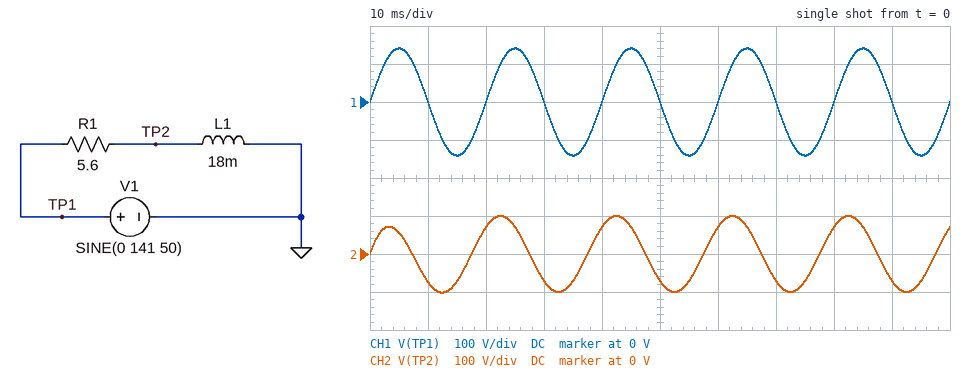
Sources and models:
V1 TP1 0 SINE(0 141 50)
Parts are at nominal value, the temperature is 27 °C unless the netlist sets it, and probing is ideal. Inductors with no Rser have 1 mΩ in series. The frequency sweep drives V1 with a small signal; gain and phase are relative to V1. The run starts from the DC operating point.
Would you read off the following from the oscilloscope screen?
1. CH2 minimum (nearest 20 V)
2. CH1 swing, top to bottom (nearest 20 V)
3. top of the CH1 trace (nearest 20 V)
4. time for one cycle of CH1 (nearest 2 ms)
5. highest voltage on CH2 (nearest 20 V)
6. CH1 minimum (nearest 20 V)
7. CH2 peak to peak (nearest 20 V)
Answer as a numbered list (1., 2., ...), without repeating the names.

1. -100 V
2. 280 V
3. 140 V
4. 20 ms
5. 100 V
6. -140 V
7. 200 V
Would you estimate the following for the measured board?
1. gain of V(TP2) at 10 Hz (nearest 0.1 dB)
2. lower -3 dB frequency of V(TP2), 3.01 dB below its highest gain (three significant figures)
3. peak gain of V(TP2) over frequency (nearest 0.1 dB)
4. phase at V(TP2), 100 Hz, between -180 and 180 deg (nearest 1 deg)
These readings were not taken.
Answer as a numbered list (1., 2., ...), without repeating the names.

1. -14.1 dB
2. 49.5 Hz
3. 0 dB
4. 26 deg
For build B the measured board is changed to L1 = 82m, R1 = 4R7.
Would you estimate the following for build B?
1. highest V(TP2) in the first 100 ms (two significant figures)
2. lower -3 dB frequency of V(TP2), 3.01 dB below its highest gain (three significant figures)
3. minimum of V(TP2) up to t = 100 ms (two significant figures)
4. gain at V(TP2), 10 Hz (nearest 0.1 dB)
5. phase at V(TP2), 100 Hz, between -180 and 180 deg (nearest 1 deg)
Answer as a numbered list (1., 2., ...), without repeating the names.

1. 140 V
2. 9.12 Hz
3. -150 V
4. -2.6 dB
5. 5 deg
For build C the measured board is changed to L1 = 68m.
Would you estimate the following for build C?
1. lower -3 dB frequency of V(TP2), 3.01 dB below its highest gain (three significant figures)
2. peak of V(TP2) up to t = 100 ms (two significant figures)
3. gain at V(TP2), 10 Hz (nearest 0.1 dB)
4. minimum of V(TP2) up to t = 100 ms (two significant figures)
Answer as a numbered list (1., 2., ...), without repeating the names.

1. 13.1 Hz
2. 140 V
3. -4.3 dB
4. -150 V
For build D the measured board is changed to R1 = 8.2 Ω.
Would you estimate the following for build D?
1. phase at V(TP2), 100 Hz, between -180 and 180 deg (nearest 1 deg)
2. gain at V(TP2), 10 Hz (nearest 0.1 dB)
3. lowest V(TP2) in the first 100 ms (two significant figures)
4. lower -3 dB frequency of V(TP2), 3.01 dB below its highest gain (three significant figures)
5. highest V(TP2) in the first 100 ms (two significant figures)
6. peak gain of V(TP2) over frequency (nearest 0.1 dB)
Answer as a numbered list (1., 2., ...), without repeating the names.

1. 36 deg
2. -17.3 dB
3. -80 V
4. 72.5 Hz
5. 80 V
6. 0 dB
